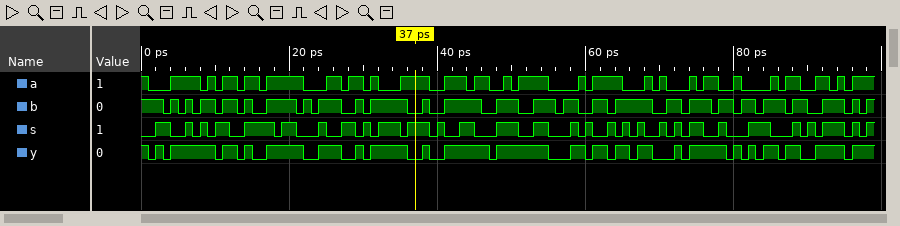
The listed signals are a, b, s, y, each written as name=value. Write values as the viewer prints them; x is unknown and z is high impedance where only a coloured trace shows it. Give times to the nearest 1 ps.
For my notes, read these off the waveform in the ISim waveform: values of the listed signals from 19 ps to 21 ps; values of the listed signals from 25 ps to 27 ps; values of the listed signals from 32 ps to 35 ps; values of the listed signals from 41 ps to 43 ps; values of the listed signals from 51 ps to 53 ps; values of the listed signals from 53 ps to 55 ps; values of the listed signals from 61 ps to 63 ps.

a=1, b=1, s=1, y=1
a=1, b=1, s=0, y=1
a=0, b=1, s=1, y=1
a=1, b=1, s=0, y=1
a=1, b=0, s=0, y=1
a=1, b=1, s=1, y=1
a=1, b=1, s=0, y=1
